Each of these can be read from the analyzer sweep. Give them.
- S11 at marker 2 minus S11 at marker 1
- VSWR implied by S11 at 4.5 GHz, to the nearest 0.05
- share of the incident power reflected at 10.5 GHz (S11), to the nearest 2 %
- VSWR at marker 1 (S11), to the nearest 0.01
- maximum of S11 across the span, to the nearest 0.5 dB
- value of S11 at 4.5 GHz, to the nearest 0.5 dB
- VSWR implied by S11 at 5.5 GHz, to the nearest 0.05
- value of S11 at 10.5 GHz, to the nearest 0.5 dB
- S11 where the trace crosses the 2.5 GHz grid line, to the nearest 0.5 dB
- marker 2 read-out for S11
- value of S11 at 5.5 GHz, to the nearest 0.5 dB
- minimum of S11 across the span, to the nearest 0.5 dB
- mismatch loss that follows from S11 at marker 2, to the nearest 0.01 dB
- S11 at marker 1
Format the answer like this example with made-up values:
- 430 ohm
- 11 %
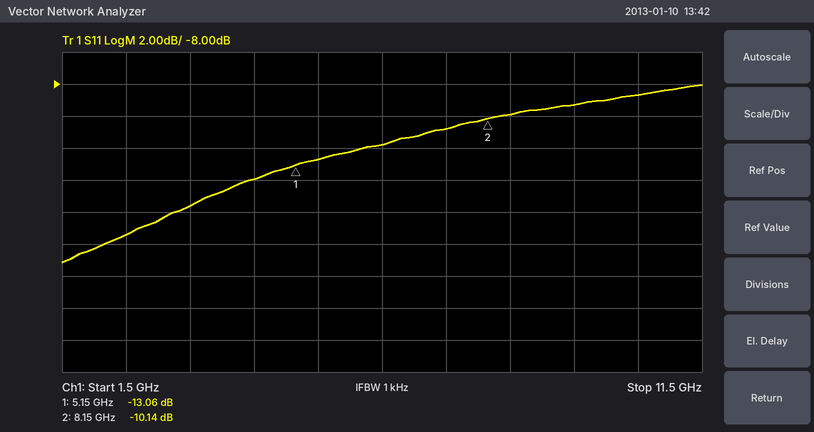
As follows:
- 2.92 dB
- 1.50
- 14 %
- 1.57
- -8.0 dB
- -14.0 dB
- 1.60
- -8.5 dB
- -17.5 dB
- -10.14 dB
- -12.5 dB
- -19.0 dB
- 0.44 dB
- -13.06 dB
